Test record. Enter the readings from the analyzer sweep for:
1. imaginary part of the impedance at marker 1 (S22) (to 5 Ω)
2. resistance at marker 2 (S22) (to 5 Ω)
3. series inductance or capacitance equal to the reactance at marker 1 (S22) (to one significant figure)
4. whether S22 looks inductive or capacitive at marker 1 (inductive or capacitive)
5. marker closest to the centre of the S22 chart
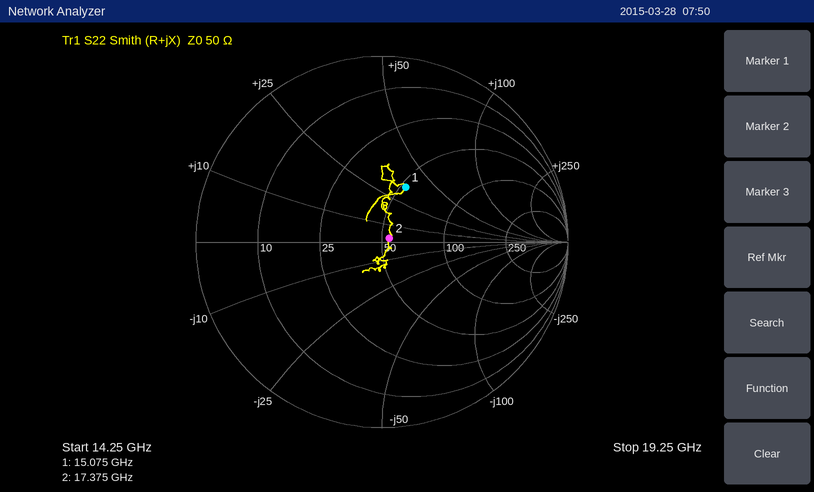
+35 Ω
55 Ω
400 pH
inductive
marker 2
